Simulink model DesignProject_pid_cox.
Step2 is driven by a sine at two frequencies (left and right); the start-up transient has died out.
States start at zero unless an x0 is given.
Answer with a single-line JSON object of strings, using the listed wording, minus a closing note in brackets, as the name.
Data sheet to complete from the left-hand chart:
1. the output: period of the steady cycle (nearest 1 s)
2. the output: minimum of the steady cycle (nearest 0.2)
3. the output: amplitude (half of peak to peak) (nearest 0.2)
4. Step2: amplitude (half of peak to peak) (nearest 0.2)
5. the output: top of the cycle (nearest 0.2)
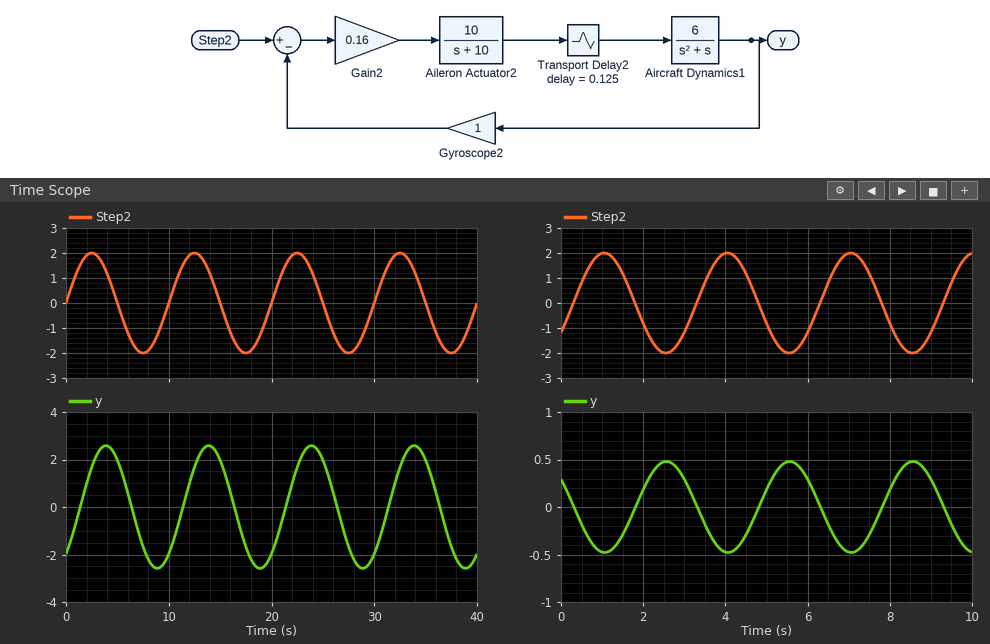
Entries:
{"the output: period of the steady cycle": "10 s", "the output: minimum of the steady cycle": "-2.6", "the output: amplitude (half of peak to peak)": "2.6", "Step2: amplitude (half of peak to peak)": "2.0", "the output: top of the cycle": "2.6"}
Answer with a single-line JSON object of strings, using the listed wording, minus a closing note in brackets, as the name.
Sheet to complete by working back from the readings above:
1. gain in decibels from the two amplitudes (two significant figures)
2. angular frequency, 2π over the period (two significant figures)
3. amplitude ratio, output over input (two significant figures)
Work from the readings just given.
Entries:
{"gain in decibels from the two amplitudes": "2.3 dB", "angular frequency, 2π over the period": "0.63 rad/s", "amplitude ratio, output over input": "1.3"}
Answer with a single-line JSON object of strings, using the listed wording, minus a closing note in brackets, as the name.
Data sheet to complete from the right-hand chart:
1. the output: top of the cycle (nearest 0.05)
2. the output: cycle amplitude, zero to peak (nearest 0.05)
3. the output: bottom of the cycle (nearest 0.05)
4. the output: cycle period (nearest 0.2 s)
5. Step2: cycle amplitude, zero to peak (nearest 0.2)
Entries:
{"the output: top of the cycle": "0.50", "the output: cycle amplitude, zero to peak": "0.50", "the output: bottom of the cycle": "-0.50", "the output: cycle period": "3.0 s", "Step2: cycle amplitude, zero to peak": "2.0"}
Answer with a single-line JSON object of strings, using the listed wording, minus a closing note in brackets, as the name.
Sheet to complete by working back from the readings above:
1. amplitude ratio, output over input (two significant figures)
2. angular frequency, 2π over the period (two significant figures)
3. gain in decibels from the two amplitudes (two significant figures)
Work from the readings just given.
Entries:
{"amplitude ratio, output over input": "0.25", "angular frequency, 2π over the period": "2.1 rad/s", "gain in decibels from the two amplitudes": "-12 dB"}
